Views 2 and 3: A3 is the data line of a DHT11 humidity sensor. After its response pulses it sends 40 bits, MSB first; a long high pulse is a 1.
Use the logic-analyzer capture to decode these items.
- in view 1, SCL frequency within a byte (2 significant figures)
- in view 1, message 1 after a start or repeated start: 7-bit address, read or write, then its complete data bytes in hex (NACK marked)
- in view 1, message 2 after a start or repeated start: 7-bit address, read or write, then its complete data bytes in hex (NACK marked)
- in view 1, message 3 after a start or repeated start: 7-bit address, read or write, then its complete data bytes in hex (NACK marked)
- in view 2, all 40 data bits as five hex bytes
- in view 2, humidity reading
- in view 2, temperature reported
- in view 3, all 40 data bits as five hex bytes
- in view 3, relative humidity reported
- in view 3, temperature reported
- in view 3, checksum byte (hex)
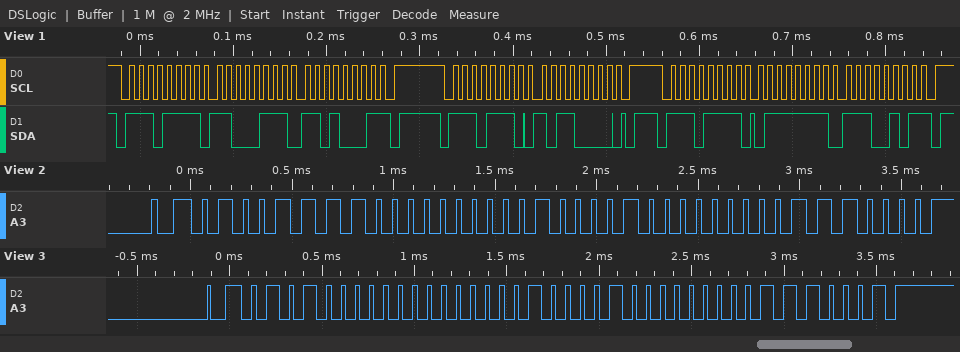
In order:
100 kHz
0x77 read: C7 D1 NACK
0x77 write: B0
0x77 read: 7F E5 NACK
4F 00 21 00 70
79 %
33.0 °C
50 00 21 00 71
80 %
33.0 °C
0x71
